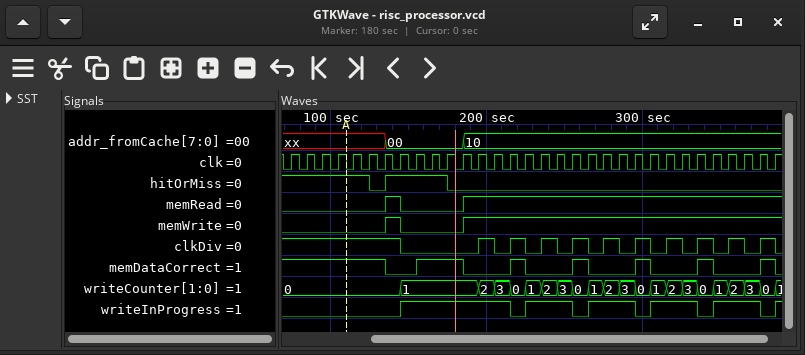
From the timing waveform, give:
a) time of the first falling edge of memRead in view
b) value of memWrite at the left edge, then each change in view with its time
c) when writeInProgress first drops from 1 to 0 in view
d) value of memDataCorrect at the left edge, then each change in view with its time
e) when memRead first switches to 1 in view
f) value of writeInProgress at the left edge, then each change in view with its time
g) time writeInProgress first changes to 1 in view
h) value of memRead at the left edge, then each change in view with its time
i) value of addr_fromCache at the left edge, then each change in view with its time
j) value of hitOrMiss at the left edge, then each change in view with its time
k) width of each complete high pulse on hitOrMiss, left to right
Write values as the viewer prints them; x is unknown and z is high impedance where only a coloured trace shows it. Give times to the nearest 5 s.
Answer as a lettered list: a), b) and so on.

a) 145 s
b) 0, 1 at 135 s, 0 at 145 s, 1 at 185 s
c) 215 s
d) 1, 0 at 135 s, 1 at 155 s, 0 at 185 s, 1 at 215 s, 0 at 225 s, 1 at 255 s, 0 at 265 s, 1 at 295 s, 0 at 305 s, 1 at 335 s, 0 at 345 s, 1 at 375 s, 0 at 385 s
e) 135 s
f) 0, 1 at 145 s, 0 at 215 s, 1 at 225 s, 0 at 255 s, 1 at 265 s, 0 at 295 s, 1 at 305 s, 0 at 335 s, 1 at 345 s, 0 at 375 s, 1 at 385 s
g) 145 s
h) 0, 1 at 135 s, 0 at 145 s, 1 at 185 s
i) xx, 00 at 135 s, 10 at 185 s
j) 1, 0 at 125 s, 1 at 135 s, 0 at 175 s
k) 40 s
